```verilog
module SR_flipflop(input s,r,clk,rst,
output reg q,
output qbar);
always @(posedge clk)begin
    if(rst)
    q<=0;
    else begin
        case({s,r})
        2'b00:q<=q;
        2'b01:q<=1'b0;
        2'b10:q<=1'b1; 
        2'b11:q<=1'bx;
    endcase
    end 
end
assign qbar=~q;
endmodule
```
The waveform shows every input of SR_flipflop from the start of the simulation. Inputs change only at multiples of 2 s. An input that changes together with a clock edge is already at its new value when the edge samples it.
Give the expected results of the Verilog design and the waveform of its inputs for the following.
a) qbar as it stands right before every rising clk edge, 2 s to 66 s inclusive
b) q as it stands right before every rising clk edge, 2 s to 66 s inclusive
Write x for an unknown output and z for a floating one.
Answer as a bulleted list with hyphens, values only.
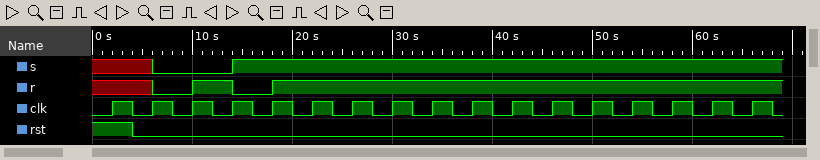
- x 1 1 1 0 x x x x x x x x x x x x
- x 0 0 0 1 x x x x x x x x x x x x
